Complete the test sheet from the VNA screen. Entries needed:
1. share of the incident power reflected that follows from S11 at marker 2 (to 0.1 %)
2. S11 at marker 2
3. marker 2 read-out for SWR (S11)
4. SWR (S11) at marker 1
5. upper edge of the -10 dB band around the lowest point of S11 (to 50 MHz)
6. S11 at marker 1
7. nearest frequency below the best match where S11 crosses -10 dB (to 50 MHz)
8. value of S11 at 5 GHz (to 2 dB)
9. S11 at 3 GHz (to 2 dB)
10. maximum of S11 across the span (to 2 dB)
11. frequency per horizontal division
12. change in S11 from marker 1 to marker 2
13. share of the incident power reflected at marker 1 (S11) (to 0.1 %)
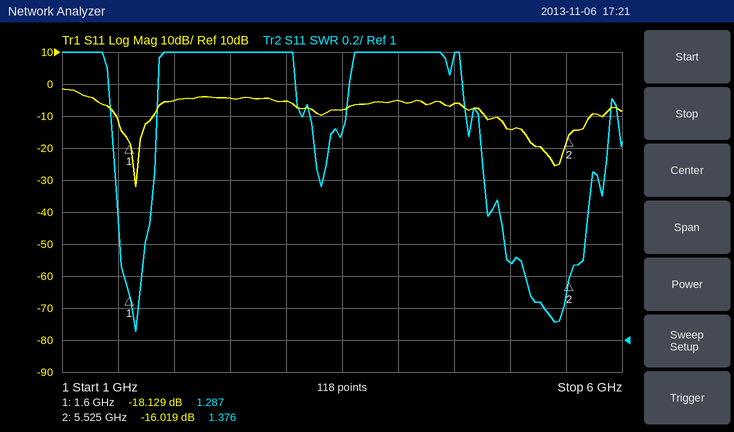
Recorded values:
2.5 %
-16.019 dB
1.376
1.287
1.80 GHz
-18.129 dB
1.50 GHz
-14 dB
-6 dB
-2 dB
500 MHz
2.110 dB
1.5 %
